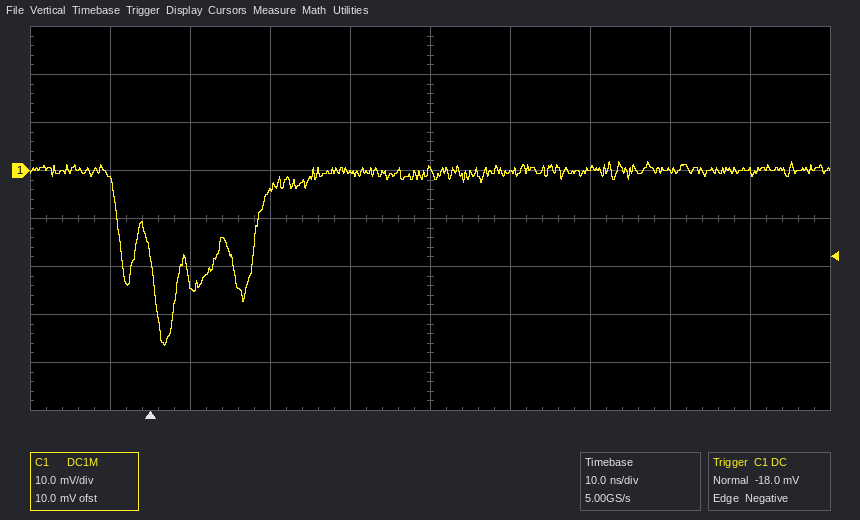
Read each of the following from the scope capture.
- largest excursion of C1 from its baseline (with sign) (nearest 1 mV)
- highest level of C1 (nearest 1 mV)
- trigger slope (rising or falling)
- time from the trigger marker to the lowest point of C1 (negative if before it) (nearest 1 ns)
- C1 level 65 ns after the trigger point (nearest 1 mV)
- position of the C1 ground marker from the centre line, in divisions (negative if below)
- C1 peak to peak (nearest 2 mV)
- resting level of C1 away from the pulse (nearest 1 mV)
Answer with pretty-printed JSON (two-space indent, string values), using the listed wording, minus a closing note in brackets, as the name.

{
  "largest excursion of C1 from its baseline (with sign)": "-36 mV",
  "highest level of C1": "2 mV",
  "trigger slope": "falling",
  "time from the trigger marker to the lowest point of C1 (negative if before it)": "+2 ns",
  "C1 level 65 ns after the trigger point": "0 mV",
  "position of the C1 ground marker from the centre line, in divisions": "+1.0 div",
  "C1 peak to peak": "38 mV",
  "resting level of C1 away from the pulse": "0 mV"
}
